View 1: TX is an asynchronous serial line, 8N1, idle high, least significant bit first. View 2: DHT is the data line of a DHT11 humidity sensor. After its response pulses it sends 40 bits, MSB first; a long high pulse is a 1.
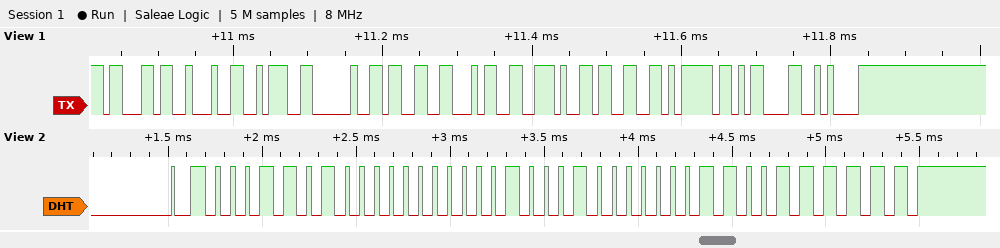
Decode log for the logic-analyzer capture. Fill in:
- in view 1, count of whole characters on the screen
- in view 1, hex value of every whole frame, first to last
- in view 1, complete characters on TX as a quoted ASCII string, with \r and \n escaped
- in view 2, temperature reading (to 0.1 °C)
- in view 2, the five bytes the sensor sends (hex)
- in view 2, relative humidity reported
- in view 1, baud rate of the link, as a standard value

11
63 22 3A 20 33 34 2E 33 7D 0D 0A
"c\": 34.3}\r\n"
34.3 °C
1A 00 22 03 3F
26 %
115200 baud
